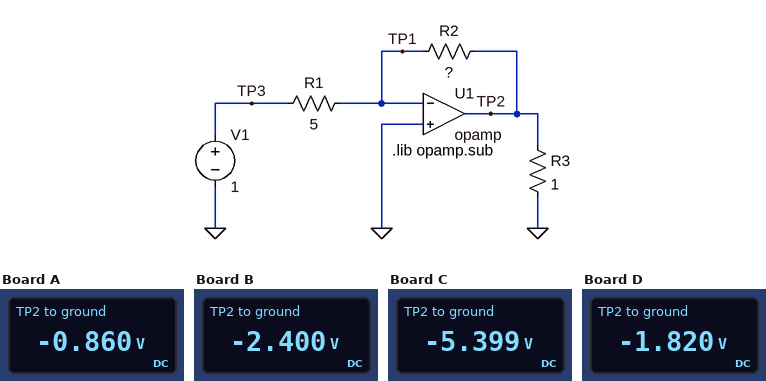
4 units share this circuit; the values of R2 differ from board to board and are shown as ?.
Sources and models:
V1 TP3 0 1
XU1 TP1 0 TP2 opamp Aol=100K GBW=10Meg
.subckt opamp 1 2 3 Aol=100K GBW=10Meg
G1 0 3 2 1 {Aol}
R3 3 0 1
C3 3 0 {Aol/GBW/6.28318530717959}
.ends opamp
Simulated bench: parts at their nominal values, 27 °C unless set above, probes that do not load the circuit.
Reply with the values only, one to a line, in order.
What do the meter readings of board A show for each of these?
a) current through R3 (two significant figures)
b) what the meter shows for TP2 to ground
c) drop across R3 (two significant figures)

860 mA
-0.860 V
860 mV
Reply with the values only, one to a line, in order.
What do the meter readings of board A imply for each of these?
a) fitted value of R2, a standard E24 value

4.3 Ω
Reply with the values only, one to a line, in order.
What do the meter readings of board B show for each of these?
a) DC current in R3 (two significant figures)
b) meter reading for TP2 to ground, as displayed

2.4 A
-2.400 V
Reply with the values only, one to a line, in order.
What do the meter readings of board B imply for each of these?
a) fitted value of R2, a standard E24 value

12 Ω
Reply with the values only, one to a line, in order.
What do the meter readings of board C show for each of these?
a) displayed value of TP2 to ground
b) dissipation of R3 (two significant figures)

-5.399 V
29 W
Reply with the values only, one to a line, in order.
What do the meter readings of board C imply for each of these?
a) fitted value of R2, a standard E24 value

27 Ω
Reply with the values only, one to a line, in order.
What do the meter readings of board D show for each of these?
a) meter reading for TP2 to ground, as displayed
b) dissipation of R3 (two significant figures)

-1.820 V
3.3 W
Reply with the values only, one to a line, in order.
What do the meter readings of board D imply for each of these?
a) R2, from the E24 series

9.1 Ω
